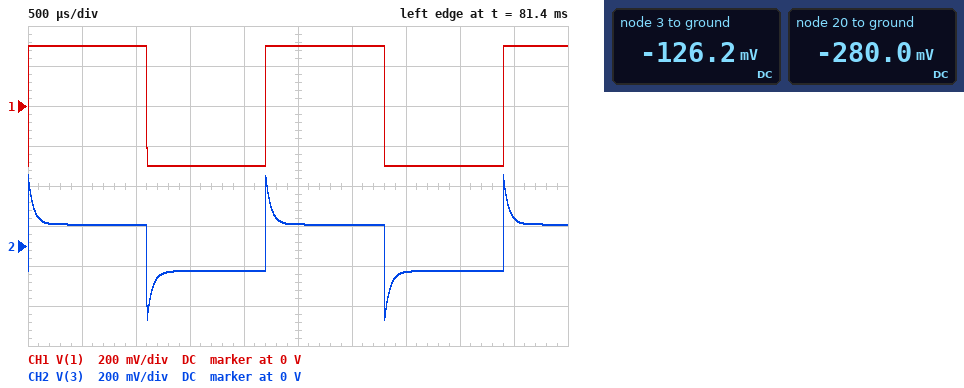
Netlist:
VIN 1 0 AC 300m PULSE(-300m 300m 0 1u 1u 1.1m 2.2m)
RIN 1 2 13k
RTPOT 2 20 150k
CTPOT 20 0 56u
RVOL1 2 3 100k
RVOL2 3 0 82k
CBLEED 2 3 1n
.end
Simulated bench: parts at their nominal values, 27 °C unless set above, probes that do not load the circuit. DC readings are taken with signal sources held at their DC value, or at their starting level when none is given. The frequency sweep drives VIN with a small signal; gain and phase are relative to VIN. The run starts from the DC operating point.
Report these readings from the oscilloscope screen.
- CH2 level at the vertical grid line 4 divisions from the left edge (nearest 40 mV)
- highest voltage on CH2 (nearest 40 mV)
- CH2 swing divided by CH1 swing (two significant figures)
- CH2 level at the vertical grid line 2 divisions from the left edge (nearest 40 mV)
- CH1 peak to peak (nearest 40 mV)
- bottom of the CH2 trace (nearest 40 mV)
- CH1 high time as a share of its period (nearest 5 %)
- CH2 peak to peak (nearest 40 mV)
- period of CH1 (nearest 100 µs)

-120 mV
360 mV
1.2
120 mV
600 mV
-360 mV
50 %
720 mV
2.2 ms
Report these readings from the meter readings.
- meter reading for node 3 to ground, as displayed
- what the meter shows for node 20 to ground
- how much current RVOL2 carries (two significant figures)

-126.2 mV
-280.0 mV
1.5 µA
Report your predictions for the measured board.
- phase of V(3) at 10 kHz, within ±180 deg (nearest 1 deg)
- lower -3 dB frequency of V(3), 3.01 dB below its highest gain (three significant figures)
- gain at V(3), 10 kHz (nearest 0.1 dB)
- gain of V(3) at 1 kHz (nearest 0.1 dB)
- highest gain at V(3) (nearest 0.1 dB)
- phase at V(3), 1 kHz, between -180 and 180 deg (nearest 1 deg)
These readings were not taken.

9 deg
2.39 kHz
-2.2 dB
-7.1 dB
-1.9 dB
15 deg
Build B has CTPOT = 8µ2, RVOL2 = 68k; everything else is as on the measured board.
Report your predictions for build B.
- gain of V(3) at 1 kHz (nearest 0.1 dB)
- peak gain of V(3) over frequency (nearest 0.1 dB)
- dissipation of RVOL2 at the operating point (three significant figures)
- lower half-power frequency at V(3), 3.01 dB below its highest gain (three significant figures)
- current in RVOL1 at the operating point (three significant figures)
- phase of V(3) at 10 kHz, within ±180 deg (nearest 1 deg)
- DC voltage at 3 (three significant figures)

-8.1 dB
-2.1 dB
187 nW
2.79 kHz
1.66 µA
11 deg
-113 mV
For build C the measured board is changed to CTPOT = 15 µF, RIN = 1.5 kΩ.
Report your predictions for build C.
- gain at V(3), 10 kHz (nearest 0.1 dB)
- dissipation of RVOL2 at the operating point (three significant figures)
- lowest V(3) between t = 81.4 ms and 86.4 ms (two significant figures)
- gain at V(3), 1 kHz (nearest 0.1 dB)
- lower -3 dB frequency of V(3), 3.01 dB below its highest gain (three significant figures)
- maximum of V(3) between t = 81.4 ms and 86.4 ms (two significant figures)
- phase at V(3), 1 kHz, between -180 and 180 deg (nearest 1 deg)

-0.6 dB
219 nW
-450 mV
-6.0 dB
2.68 kHz
450 mV
16 deg
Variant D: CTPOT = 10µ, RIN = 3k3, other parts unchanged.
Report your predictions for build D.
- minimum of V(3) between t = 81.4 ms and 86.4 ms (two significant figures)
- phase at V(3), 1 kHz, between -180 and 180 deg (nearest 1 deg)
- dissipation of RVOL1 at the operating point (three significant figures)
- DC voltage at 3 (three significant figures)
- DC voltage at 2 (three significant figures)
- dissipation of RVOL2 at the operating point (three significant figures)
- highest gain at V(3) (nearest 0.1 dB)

-430 mV
16 deg
262 nW
-133 mV
-295 mV
215 nW
-0.5 dB
